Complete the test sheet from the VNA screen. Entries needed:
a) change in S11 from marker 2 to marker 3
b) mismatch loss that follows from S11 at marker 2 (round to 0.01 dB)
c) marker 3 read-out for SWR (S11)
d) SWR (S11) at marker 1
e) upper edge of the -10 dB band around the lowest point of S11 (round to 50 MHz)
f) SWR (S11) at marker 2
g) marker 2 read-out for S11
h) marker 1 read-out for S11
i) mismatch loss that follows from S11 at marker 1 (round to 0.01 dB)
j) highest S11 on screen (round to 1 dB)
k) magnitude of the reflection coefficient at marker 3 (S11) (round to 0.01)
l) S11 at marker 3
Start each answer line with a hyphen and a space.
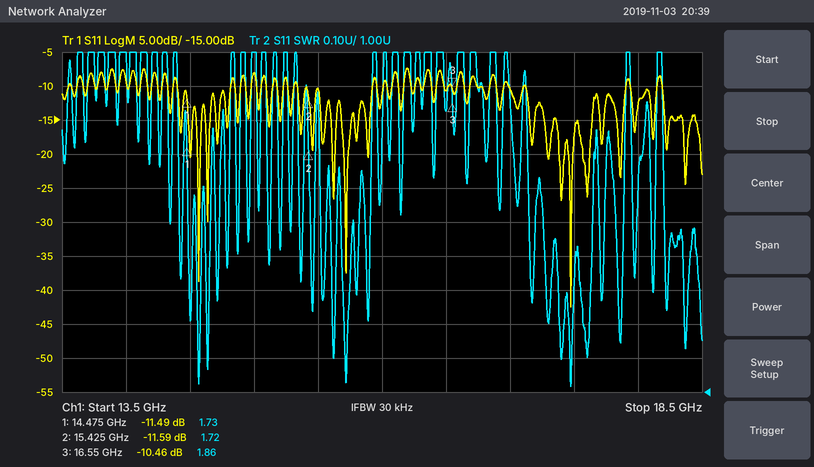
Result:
- 1.13 dB
- 0.31 dB
- 1.86
- 1.73
- 17.90 GHz
- 1.72
- -11.59 dB
- -11.49 dB
- 0.32 dB
- -7 dB
- 0.30
- -10.46 dB
